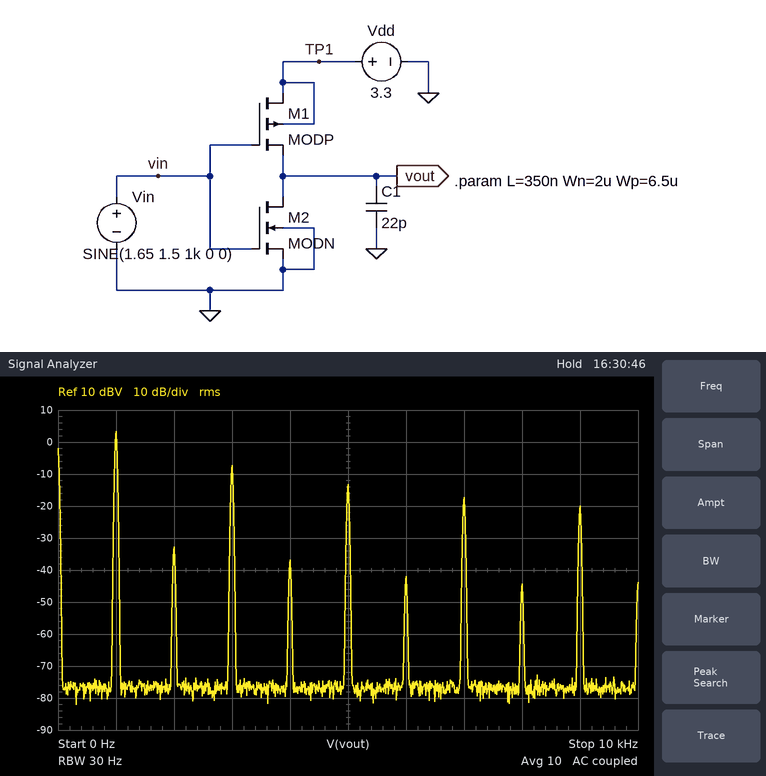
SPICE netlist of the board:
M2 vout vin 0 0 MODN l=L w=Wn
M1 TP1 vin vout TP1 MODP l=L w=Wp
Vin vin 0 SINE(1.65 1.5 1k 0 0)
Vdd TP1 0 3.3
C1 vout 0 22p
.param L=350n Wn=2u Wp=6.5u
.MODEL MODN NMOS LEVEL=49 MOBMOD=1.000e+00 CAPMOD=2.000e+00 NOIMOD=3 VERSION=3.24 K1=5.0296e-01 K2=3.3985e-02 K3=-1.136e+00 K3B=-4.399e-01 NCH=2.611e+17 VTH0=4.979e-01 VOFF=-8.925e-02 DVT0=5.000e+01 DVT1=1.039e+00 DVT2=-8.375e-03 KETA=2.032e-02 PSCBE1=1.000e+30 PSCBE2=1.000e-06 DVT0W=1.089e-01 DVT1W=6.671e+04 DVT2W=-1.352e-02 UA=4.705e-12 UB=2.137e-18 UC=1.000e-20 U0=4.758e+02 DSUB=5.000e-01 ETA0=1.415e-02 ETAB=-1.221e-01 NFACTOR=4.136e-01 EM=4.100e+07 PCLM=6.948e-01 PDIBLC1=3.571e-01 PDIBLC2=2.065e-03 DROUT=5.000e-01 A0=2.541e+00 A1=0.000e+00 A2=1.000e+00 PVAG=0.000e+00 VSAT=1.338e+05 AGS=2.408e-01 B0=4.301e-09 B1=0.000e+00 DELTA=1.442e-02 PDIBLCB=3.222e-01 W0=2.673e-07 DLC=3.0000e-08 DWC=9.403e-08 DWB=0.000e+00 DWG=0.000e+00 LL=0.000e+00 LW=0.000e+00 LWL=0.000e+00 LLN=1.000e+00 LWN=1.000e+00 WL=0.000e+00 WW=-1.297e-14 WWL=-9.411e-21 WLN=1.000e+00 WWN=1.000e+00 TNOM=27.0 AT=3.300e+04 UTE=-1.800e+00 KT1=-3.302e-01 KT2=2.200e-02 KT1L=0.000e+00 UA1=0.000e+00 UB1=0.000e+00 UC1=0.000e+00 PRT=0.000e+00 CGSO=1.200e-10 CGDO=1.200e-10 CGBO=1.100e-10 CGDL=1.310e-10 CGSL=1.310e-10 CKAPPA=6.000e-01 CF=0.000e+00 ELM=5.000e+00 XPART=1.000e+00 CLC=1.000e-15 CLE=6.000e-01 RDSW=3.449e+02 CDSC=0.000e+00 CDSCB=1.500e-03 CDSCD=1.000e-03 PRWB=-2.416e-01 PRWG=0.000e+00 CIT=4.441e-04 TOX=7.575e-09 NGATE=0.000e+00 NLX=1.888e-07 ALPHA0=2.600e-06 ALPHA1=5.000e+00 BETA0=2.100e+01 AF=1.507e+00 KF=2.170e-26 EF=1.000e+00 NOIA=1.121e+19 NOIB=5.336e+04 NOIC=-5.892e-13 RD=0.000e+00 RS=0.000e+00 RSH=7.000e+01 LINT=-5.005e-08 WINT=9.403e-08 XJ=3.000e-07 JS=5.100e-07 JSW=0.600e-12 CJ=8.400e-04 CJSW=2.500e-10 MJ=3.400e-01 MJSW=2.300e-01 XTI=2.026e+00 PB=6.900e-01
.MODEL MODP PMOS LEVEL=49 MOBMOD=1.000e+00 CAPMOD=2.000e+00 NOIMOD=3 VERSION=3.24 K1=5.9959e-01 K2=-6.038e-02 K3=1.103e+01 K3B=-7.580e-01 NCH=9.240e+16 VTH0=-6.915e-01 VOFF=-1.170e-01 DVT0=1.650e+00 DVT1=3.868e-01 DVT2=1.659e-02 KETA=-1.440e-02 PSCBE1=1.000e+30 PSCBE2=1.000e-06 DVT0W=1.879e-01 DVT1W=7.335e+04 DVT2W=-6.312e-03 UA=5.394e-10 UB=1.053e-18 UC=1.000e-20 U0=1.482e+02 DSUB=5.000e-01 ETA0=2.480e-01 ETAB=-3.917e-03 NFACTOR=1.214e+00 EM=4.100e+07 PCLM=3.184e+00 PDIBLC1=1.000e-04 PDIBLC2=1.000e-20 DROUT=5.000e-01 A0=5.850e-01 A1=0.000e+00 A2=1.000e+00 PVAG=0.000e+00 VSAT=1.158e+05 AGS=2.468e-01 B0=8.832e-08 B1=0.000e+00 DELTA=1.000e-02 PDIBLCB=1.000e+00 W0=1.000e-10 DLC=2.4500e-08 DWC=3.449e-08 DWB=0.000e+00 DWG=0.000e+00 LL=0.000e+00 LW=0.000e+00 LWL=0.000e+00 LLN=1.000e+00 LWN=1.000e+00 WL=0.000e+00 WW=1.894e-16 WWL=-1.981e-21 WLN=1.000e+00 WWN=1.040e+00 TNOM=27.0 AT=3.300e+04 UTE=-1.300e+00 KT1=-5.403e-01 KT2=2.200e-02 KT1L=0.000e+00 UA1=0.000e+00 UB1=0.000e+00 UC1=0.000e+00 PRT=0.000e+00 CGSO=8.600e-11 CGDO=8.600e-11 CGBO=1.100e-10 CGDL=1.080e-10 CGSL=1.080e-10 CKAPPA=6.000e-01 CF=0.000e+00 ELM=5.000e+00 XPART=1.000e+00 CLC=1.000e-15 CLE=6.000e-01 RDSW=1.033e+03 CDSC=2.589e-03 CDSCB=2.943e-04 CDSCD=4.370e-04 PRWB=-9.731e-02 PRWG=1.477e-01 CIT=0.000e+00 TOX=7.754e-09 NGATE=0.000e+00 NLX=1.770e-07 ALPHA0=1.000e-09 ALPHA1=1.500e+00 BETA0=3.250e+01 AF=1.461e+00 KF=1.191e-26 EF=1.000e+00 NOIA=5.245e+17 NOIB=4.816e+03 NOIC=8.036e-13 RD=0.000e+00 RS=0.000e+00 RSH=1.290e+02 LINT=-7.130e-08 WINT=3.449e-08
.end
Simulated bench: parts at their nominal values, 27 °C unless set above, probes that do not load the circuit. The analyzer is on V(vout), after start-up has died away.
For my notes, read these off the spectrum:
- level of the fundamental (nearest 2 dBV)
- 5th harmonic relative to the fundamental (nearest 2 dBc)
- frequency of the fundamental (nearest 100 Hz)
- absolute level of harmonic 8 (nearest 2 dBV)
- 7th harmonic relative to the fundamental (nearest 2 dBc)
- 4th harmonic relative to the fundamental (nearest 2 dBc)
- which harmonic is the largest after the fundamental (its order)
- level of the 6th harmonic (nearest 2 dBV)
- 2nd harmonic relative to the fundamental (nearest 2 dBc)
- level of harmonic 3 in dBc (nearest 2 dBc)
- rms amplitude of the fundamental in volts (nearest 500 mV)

4 dBV
-16 dBc
1.0 kHz
-44 dBV
-20 dBc
-40 dBc
3
-42 dBV
-36 dBc
-10 dBc
1.5 V
